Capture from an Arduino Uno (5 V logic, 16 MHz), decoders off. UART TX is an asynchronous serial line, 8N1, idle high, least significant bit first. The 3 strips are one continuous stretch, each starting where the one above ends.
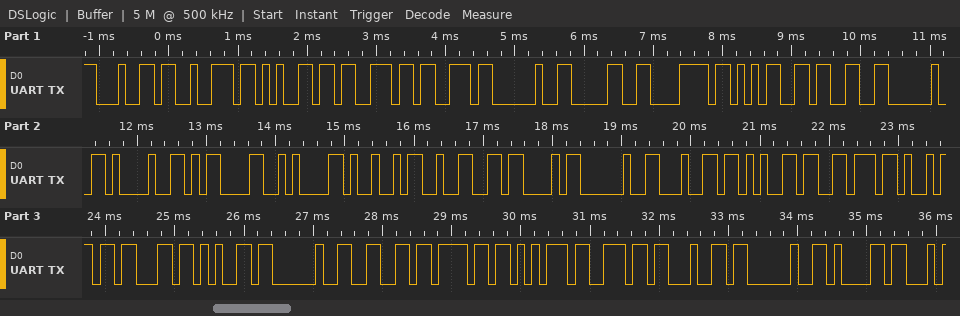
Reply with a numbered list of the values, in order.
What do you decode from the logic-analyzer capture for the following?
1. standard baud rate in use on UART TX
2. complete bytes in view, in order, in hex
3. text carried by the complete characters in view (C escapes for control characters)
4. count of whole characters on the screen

1. 9600 baud
2. 64 72 65 73 73 20 30 78 35 33 20 21 0D 0A 49 32 43 20 64 65 76 69 63 65 20 66 6F 75 6E 64 20 61
3. "dress 0x53 !\r\nI2C device found a"
4. 32
